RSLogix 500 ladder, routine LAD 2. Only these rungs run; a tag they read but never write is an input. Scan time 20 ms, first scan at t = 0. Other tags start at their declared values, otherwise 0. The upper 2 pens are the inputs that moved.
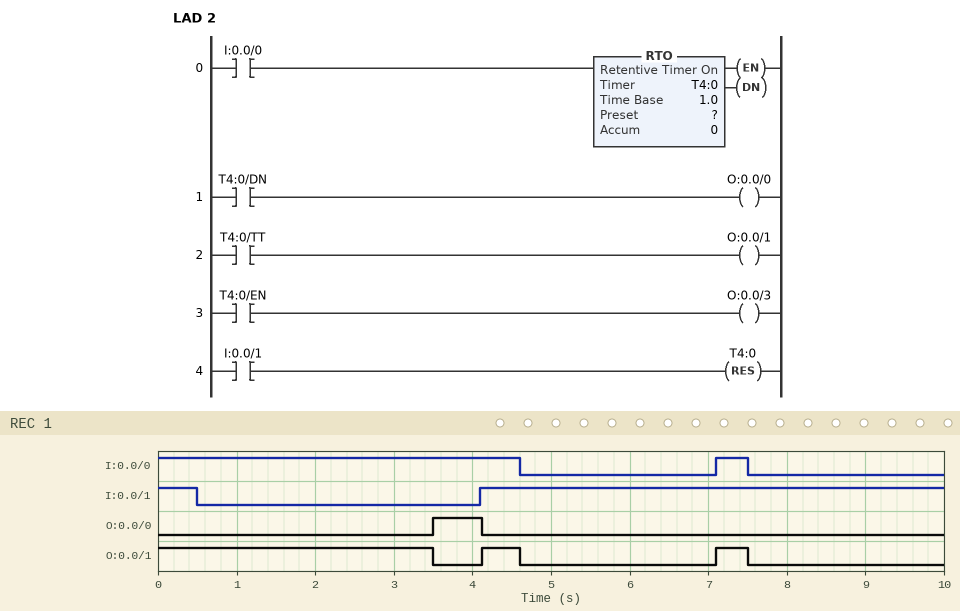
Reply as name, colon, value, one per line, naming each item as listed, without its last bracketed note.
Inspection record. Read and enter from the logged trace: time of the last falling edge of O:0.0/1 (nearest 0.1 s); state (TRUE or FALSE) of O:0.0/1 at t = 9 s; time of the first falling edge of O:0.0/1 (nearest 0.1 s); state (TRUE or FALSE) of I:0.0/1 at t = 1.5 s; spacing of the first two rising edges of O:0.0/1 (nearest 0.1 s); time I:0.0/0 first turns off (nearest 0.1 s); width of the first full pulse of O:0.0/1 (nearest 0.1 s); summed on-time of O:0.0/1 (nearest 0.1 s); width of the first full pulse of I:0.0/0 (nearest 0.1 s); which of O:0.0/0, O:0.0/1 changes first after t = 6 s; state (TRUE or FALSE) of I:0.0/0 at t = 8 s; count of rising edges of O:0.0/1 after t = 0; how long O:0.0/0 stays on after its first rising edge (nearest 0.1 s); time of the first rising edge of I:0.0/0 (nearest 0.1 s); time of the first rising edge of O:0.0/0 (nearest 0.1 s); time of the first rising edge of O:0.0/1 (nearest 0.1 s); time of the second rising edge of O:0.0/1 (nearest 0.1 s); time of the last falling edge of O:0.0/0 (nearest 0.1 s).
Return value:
time of the last falling edge of O:0.0/1: 7.5 s
state (TRUE or FALSE) of O:0.0/1 at t = 9 s: FALSE
time of the first falling edge of O:0.0/1: 3.5 s
state (TRUE or FALSE) of I:0.0/1 at t = 1.5 s: FALSE
spacing of the first two rising edges of O:0.0/1: 3.0 s
time I:0.0/0 first turns off: 4.6 s
width of the first full pulse of O:0.0/1: 0.5 s
summed on-time of O:0.0/1: 4.4 s
width of the first full pulse of I:0.0/0: 0.4 s
which of O:0.0/0, O:0.0/1 changes first after t = 6 s: O:0.0/1
state (TRUE or FALSE) of I:0.0/0 at t = 8 s: FALSE
count of rising edges of O:0.0/1 after t = 0: 2
how long O:0.0/0 stays on after its first rising edge: 0.6 s
time of the first rising edge of I:0.0/0: 7.1 s
time of the first rising edge of O:0.0/0: 3.5 s
time of the first rising edge of O:0.0/1: 4.1 s
time of the second rising edge of O:0.0/1: 7.1 s
time of the last falling edge of O:0.0/0: 4.1 s
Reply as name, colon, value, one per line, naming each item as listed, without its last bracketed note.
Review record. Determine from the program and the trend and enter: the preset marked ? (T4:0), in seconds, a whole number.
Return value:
the preset marked ? (T4:0), in seconds, a whole number: 3 s
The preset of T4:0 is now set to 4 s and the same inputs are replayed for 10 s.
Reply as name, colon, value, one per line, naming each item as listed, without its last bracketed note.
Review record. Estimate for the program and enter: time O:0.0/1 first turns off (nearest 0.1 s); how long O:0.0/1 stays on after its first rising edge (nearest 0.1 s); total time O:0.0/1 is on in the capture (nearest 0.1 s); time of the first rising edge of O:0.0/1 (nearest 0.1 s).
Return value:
time O:0.0/1 first turns off: 4.6 s
how long O:0.0/1 stays on after its first rising edge: 0.4 s
total time O:0.0/1 is on in the capture: 5.0 s
time of the first rising edge of O:0.0/1: 7.1 s
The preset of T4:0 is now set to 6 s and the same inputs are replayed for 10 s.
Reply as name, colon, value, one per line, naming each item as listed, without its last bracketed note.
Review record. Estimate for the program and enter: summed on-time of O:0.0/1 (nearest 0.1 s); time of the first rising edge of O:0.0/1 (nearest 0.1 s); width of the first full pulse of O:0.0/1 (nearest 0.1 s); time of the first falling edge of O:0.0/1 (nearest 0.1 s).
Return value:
summed on-time of O:0.0/1: 5.0 s
time of the first rising edge of O:0.0/1: 7.1 s
width of the first full pulse of O:0.0/1: 0.4 s
time of the first falling edge of O:0.0/1: 4.6 s
